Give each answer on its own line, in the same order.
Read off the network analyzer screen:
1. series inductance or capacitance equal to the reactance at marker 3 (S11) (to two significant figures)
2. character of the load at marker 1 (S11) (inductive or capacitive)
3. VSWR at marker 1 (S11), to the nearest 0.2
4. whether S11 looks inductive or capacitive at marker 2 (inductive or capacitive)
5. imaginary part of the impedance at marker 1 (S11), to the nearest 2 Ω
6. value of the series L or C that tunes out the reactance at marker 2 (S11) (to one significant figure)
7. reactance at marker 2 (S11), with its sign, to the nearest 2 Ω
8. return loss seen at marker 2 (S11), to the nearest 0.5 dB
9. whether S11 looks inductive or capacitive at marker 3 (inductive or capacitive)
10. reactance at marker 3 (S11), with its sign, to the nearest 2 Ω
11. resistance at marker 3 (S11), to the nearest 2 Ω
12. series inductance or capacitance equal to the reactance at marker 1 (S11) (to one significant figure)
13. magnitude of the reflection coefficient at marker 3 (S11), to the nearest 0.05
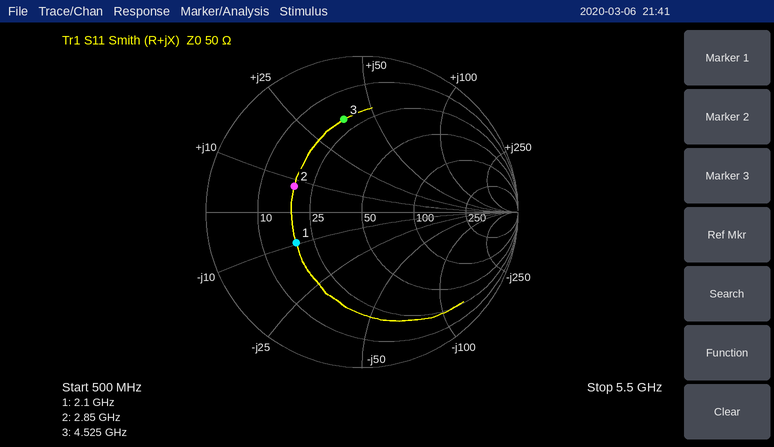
1.3 nH
capacitive
2.8
inductive
-10 Ω
7 pF
+8 Ω
6.5 dB
inductive
+38 Ω
20 Ω
8 pF
0.60
